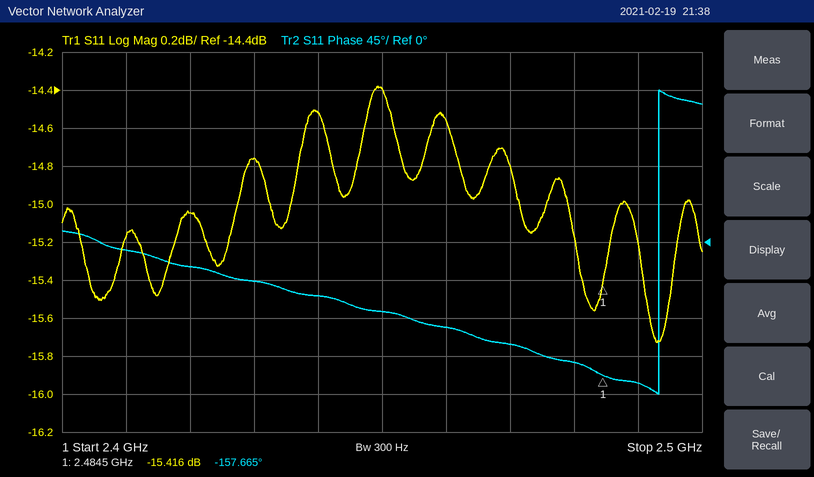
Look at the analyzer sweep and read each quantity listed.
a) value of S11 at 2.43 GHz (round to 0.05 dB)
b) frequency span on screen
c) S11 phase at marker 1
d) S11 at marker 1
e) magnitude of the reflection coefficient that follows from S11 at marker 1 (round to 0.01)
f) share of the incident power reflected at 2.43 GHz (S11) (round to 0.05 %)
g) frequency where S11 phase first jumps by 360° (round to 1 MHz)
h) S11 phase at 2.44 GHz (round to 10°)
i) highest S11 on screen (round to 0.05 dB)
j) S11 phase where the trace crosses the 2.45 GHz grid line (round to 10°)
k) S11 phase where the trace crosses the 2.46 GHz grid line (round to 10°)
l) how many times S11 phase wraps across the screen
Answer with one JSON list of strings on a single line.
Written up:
["-14.75 dB", "100 MHz", "-157.665°", "-15.416 dB", "0.17", "3.35 %", "2.493 GHz", "-60°", "-14.40 dB", "-80°", "-100°", "1"]
